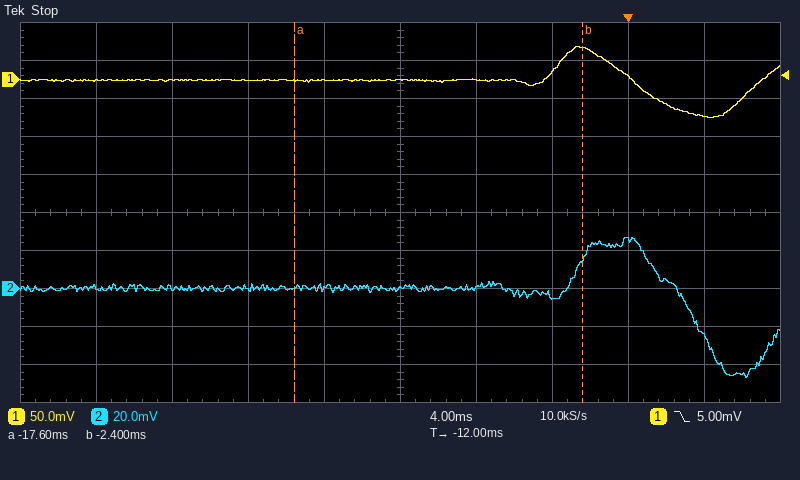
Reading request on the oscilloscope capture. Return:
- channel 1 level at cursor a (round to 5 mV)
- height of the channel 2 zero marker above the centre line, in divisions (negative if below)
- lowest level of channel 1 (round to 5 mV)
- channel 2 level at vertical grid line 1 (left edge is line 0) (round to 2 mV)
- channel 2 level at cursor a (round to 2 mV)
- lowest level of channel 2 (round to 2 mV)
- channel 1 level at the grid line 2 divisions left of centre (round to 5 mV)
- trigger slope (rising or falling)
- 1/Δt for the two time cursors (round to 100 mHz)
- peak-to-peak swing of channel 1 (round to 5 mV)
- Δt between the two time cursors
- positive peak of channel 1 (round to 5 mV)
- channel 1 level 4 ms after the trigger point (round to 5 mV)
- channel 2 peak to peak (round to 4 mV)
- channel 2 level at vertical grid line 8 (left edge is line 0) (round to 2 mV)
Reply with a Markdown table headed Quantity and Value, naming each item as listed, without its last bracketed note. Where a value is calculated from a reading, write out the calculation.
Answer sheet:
| Quantity | Value |
|---|---|
| channel 1 level at cursor a | 0 mV |
| height of the channel 2 zero marker above the centre line, in divisions | -2.0 div |
| lowest level of channel 1 | -50 mV |
| channel 2 level at vertical grid line 1 (left edge is line 0) | 0 mV |
| channel 2 level at cursor a | 0 mV |
| lowest level of channel 2 | -46 mV |
| channel 1 level at the grid line 2 divisions left of centre | 0 mV |
| trigger slope | falling |
| 1/Δt for the two time cursors | 1 / 15.2 ms ≈ 65.8 Hz |
| peak-to-peak swing of channel 1 | 45 mV − (-50 mV) = 95 mV |
| Δt between the two time cursors | -2.4 ms − (-17.6 ms) = 15.2 ms |
| positive peak of channel 1 | 45 mV |
| channel 1 level 4 ms after the trigger point | -50 mV |
| channel 2 peak to peak | 72 mV |
| channel 2 level at vertical grid line 8 (left edge is line 0) | 26 mV |
